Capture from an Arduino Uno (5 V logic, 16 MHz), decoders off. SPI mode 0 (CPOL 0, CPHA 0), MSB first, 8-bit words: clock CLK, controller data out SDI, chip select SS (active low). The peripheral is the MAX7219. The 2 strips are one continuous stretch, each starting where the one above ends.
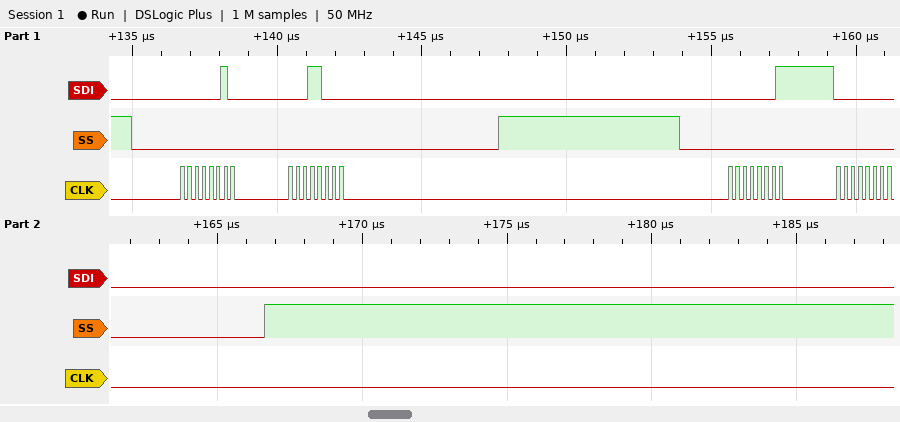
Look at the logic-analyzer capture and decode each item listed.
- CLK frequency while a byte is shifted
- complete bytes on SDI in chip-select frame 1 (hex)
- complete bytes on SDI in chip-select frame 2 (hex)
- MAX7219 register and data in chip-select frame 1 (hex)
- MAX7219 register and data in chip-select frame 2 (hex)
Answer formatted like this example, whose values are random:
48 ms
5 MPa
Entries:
4 MHz
02 18
01 00
register 0x2, data 0x18
register 0x1, data 0x00
